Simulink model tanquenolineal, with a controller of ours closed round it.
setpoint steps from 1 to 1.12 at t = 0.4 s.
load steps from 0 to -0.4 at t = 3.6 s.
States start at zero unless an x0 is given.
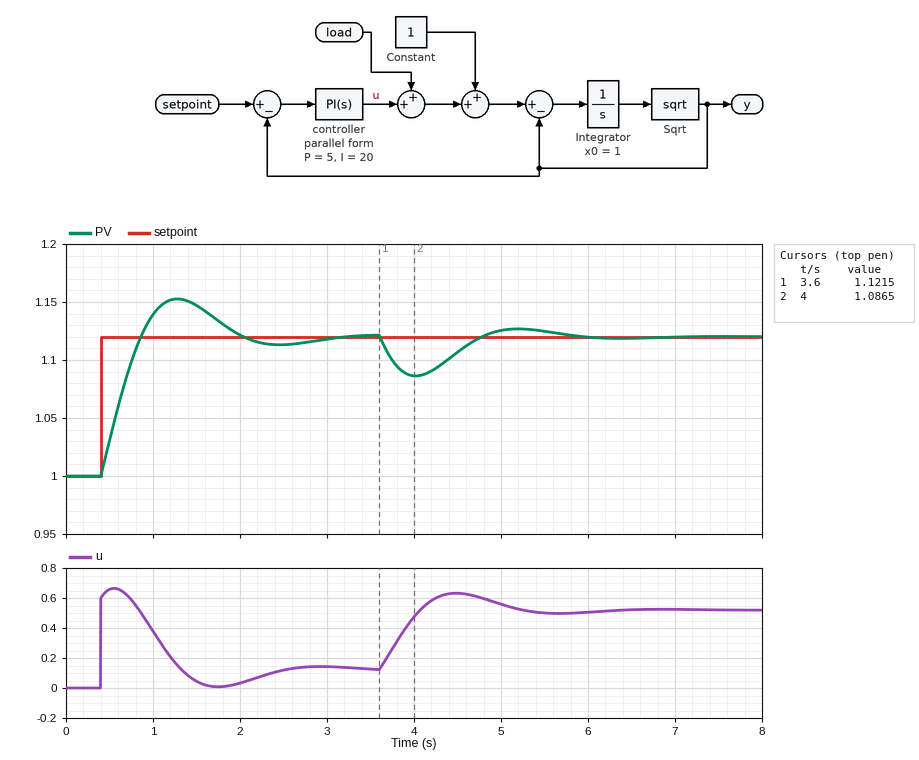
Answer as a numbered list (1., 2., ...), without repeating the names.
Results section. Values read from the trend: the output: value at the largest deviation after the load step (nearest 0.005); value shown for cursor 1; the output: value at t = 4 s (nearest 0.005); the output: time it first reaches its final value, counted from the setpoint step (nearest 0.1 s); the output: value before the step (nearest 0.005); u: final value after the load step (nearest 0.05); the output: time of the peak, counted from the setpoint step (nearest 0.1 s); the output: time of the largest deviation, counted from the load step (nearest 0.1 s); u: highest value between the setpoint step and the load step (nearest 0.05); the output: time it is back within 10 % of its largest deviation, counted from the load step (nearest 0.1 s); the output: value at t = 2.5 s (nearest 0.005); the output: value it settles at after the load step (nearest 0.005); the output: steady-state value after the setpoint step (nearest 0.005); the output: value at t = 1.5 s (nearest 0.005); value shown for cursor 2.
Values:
1. 1.085
2. 1.1215
3. 1.085
4. 0.5 s
5. 1.000
6. 0.50
7. 0.9 s
8. 0.4 s
9. 0.65
10. 2.0 s
11. 1.115
12. 1.120
13. 1.120
14. 1.145
15. 1.0865
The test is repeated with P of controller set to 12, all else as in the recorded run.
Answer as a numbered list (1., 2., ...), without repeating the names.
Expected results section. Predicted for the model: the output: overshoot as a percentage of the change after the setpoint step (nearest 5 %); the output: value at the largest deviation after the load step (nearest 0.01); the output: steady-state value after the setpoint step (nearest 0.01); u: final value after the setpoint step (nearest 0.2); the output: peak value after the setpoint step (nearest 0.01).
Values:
1. 10 %
2. 1.10
3. 1.12
4. 0.2
5. 1.13
